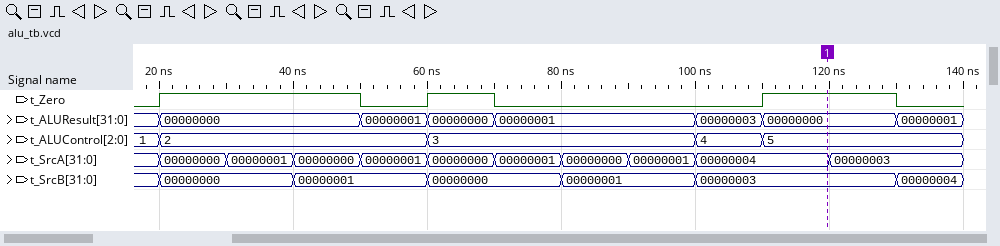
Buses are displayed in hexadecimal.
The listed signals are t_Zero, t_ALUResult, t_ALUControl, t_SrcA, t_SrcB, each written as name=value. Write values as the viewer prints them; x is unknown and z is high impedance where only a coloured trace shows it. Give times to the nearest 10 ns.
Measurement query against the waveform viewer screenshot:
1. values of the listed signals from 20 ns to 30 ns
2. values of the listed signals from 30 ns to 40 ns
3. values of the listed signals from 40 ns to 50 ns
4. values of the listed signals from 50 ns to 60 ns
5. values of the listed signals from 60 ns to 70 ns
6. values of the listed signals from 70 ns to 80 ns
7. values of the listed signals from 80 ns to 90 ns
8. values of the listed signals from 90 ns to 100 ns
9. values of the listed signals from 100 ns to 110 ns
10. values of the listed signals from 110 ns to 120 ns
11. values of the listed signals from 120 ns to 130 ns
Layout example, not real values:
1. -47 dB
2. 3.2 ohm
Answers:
1. t_Zero=1, t_ALUResult=00000000, t_ALUControl=2, t_SrcA=00000000, t_SrcB=00000000
2. t_Zero=1, t_ALUResult=00000000, t_ALUControl=2, t_SrcA=00000001, t_SrcB=00000000
3. t_Zero=1, t_ALUResult=00000000, t_ALUControl=2, t_SrcA=00000000, t_SrcB=00000001
4. t_Zero=0, t_ALUResult=00000001, t_ALUControl=2, t_SrcA=00000001, t_SrcB=00000001
5. t_Zero=1, t_ALUResult=00000000, t_ALUControl=3, t_SrcA=00000000, t_SrcB=00000000
6. t_Zero=0, t_ALUResult=00000001, t_ALUControl=3, t_SrcA=00000001, t_SrcB=00000000
7. t_Zero=0, t_ALUResult=00000001, t_ALUControl=3, t_SrcA=00000000, t_SrcB=00000001
8. t_Zero=0, t_ALUResult=00000001, t_ALUControl=3, t_SrcA=00000001, t_SrcB=00000001
9. t_Zero=0, t_ALUResult=00000003, t_ALUControl=4, t_SrcA=00000004, t_SrcB=00000003
10. t_Zero=1, t_ALUResult=00000000, t_ALUControl=5, t_SrcA=00000004, t_SrcB=00000003
11. t_Zero=1, t_ALUResult=00000000, t_ALUControl=5, t_SrcA=00000003, t_SrcB=00000003
